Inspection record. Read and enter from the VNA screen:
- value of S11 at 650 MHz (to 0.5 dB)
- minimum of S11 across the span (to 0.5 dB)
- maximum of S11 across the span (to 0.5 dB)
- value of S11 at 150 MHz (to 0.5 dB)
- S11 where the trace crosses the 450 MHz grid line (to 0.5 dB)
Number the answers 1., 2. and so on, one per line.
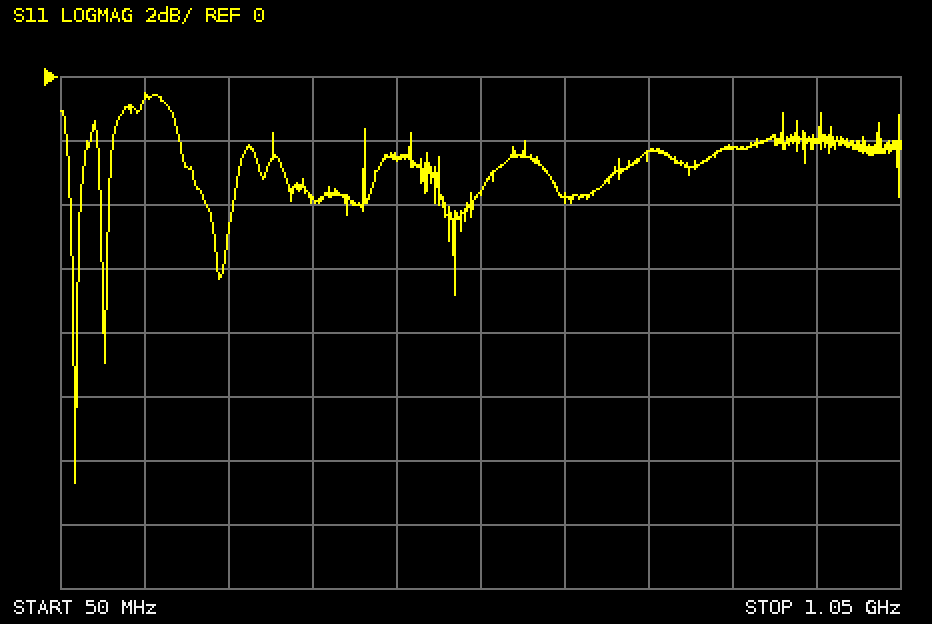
1. -4.0 dB
2. -12.5 dB
3. -0.5 dB
4. -0.5 dB
5. -2.5 dB
